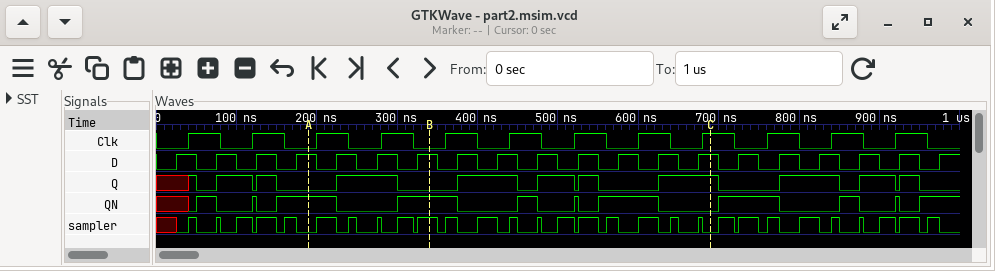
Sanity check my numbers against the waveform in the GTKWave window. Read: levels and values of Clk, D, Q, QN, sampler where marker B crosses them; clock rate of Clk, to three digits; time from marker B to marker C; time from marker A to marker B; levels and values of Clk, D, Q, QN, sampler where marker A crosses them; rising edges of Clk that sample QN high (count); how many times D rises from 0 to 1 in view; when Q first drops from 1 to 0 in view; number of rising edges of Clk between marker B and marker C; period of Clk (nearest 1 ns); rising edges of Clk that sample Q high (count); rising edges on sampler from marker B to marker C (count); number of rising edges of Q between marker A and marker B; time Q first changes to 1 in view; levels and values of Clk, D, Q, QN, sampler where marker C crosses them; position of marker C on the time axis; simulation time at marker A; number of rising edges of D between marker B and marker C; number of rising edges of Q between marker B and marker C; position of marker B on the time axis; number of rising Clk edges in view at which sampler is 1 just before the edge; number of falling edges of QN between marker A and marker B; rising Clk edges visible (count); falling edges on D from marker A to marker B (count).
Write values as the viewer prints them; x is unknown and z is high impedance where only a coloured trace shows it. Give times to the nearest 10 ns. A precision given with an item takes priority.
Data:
Clk=0, D=1, Q=0, QN=1, sampler=1
12.5 MHz
350 ns
150 ns
Clk=0, D=1, Q=0, QN=1, sampler=0
4
20
50 ns
5
80 ns
7
10
1
40 ns
Clk=1, D=1, Q=1, QN=0, sampler=0
690 ns
190 ns
7
4
340 ns
5
1
12
3
